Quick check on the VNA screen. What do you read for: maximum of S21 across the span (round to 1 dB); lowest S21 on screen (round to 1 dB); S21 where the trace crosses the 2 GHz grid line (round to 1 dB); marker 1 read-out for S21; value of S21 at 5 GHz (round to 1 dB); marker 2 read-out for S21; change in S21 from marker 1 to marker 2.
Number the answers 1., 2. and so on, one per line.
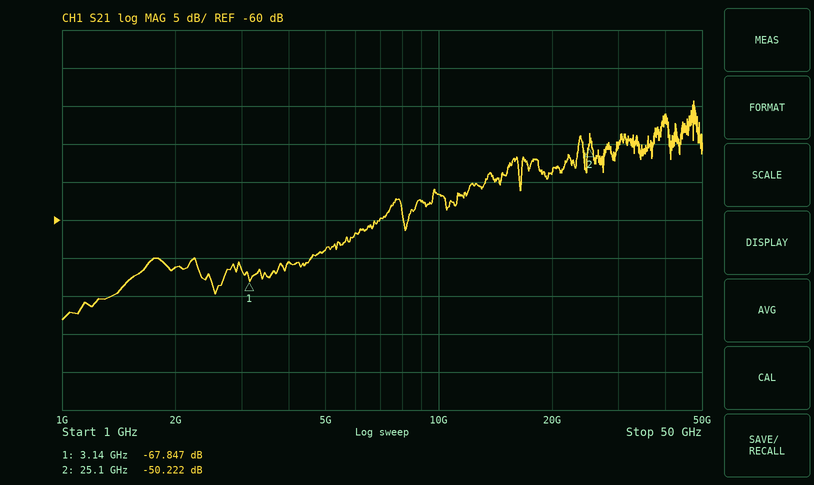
1. -44 dB
2. -73 dB
3. -66 dB
4. -67.847 dB
5. -64 dB
6. -50.222 dB
7. 17.625 dB
